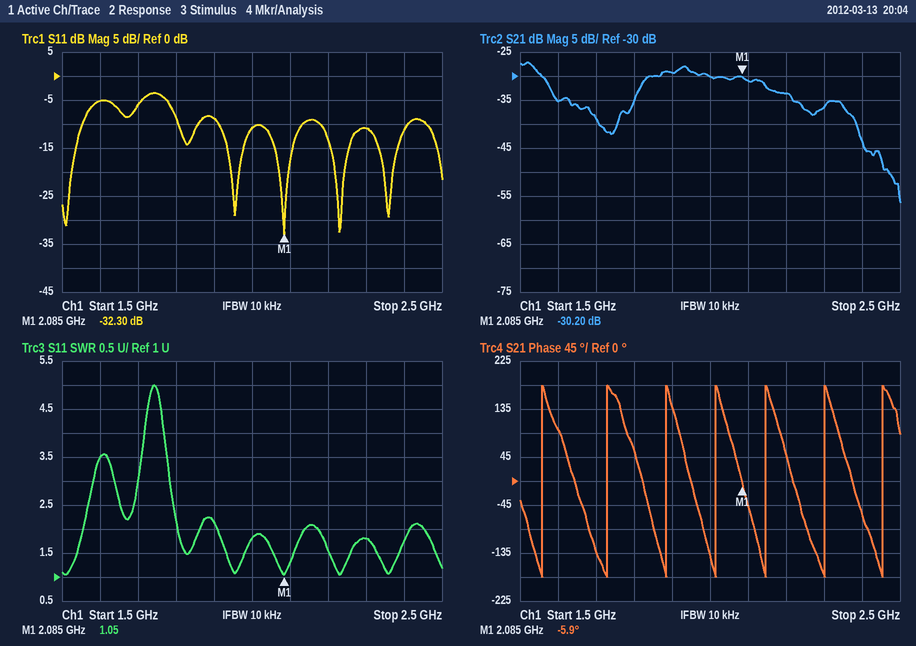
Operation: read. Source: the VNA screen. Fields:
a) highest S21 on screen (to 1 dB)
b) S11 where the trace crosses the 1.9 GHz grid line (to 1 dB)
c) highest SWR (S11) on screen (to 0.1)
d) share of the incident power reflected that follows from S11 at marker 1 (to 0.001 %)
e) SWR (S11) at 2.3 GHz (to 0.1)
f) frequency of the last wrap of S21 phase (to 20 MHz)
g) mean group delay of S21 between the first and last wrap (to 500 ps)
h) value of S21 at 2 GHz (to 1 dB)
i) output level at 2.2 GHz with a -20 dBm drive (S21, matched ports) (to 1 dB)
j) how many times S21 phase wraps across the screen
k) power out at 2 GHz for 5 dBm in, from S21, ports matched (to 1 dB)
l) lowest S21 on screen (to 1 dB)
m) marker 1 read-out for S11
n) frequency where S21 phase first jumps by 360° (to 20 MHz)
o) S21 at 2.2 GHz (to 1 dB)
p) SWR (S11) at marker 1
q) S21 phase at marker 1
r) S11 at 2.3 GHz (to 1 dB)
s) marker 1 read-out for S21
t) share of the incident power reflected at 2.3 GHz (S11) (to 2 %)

-27 dB
-9 dB
5.0
0.059 %
1.8
2.46 GHz
6.5 ns
-30 dB
-54 dBm
7
-25 dBm
-56 dB
-32.30 dB
1.56 GHz
-34 dB
1.05
-5.9°
-11 dB
-30.20 dB
8 %
